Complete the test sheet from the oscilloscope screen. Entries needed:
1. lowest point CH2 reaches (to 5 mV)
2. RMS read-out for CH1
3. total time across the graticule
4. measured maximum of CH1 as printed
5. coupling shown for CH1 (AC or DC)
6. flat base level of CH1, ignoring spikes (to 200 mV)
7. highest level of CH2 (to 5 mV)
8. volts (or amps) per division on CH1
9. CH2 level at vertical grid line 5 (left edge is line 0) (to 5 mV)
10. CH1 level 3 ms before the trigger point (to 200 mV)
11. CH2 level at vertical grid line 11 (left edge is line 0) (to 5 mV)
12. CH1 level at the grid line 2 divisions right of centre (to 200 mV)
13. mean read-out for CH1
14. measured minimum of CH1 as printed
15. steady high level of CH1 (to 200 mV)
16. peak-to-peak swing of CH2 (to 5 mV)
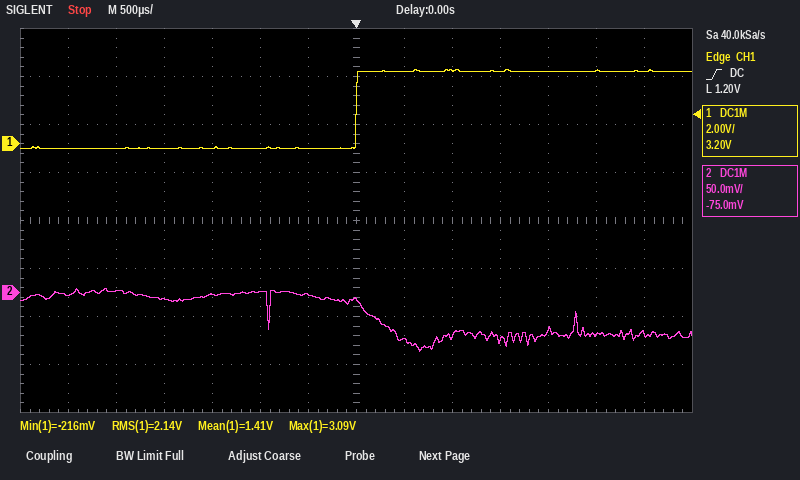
-60 mV
2.14 V
7 ms
3.09 V
DC
-200 mV
5 mV
2 V
0 mV
-200 mV
-40 mV
3.0 V
1.41 V
-216 mV
3.0 V
65 mV
